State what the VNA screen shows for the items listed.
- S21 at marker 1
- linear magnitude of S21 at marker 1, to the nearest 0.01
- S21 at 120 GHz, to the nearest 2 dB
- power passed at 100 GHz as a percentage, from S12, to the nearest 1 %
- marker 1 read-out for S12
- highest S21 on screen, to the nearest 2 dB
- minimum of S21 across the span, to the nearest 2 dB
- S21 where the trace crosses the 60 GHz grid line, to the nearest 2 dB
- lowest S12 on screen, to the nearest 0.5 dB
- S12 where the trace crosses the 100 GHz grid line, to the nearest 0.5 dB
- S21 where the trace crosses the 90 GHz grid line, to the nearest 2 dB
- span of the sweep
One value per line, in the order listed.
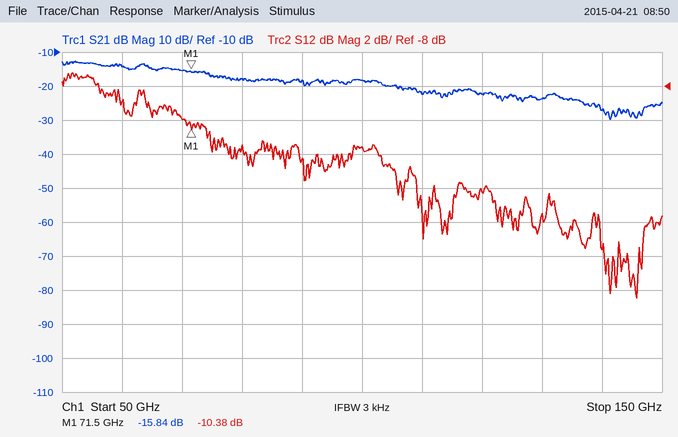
-15.84 dB
0.16
-22 dB
7 %
-10.38 dB
-12 dB
-30 dB
-14 dB
-20.5 dB
-11.5 dB
-18 dB
100 GHz
